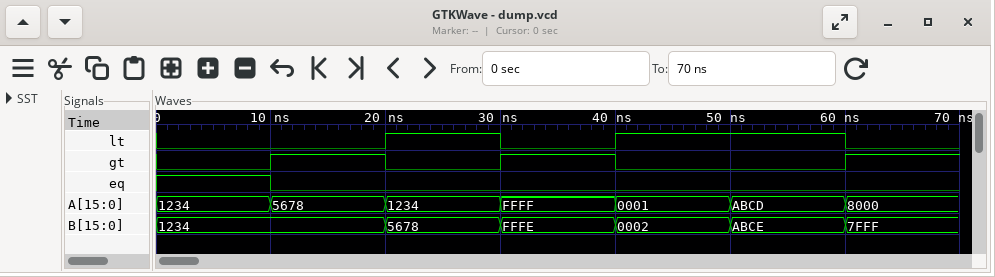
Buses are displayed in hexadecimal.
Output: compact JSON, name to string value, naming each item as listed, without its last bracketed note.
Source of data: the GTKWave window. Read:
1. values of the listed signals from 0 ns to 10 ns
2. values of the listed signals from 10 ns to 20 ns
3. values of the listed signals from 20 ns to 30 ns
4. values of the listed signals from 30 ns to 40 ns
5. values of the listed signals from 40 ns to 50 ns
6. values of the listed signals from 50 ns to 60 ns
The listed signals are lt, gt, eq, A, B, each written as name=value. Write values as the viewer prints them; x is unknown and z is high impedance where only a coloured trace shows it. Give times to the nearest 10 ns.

{"values of the listed signals from 0 ns to 10 ns": "lt=0, gt=0, eq=1, A=1234, B=1234", "values of the listed signals from 10 ns to 20 ns": "lt=0, gt=1, eq=0, A=5678, B=1234", "values of the listed signals from 20 ns to 30 ns": "lt=1, gt=0, eq=0, A=1234, B=5678", "values of the listed signals from 30 ns to 40 ns": "lt=0, gt=1, eq=0, A=FFFF, B=FFFE", "values of the listed signals from 40 ns to 50 ns": "lt=1, gt=0, eq=0, A=0001, B=0002", "values of the listed signals from 50 ns to 60 ns": "lt=1, gt=0, eq=0, A=ABCD, B=ABCE"}
